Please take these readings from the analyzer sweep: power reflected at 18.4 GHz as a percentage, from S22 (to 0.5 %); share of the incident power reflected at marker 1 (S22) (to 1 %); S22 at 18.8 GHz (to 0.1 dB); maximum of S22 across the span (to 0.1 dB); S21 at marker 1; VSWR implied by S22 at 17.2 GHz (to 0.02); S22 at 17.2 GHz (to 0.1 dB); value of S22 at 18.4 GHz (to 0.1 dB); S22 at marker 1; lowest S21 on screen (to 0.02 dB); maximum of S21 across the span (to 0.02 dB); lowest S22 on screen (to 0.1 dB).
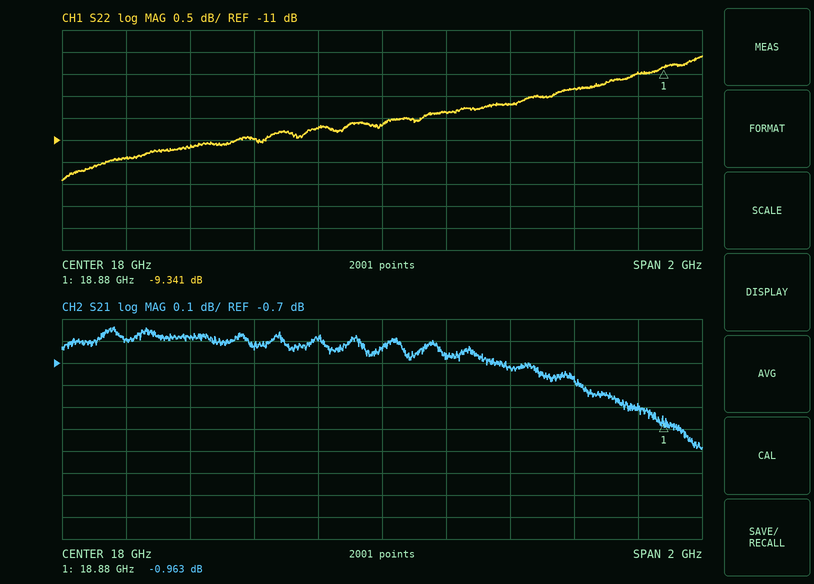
9.5 %
12 %
-9.5 dB
-9.1 dB
-0.963 dB
1.74
-11.4 dB
-10.2 dB
-9.341 dB
-1.10 dB
-0.54 dB
-11.9 dB
